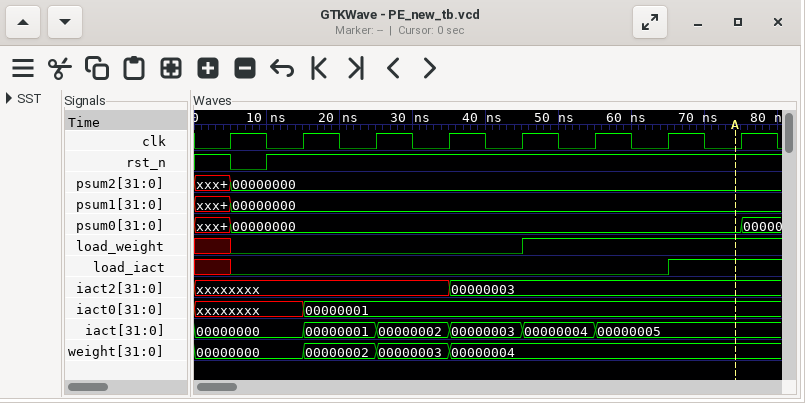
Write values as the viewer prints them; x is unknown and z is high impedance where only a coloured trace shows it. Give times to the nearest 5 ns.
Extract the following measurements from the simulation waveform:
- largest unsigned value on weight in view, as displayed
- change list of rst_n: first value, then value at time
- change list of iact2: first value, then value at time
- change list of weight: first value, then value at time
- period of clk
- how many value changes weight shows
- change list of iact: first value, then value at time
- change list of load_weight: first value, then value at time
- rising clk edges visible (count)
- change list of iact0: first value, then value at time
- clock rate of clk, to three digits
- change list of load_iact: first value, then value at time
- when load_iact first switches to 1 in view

00000004
1, 0 at 5 ns, 1 at 10 ns
xxxxxxxx, 00000003 at 35 ns
00000000, 00000002 at 15 ns, 00000003 at 25 ns, 00000004 at 35 ns
10 ns
3
00000000, 00000001 at 15 ns, 00000002 at 25 ns, 00000003 at 35 ns, 00000004 at 45 ns, 00000005 at 55 ns
x, 0 at 5 ns, 1 at 45 ns
8
xxxxxxxx, 00000001 at 15 ns
100 MHz
x, 0 at 5 ns, 1 at 65 ns
65 ns
